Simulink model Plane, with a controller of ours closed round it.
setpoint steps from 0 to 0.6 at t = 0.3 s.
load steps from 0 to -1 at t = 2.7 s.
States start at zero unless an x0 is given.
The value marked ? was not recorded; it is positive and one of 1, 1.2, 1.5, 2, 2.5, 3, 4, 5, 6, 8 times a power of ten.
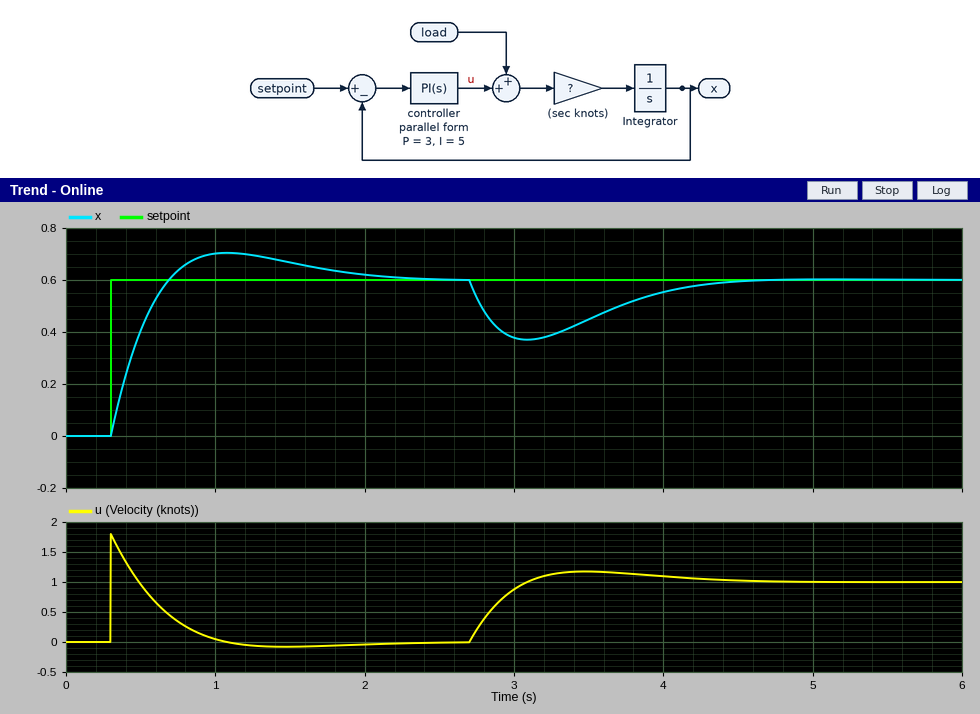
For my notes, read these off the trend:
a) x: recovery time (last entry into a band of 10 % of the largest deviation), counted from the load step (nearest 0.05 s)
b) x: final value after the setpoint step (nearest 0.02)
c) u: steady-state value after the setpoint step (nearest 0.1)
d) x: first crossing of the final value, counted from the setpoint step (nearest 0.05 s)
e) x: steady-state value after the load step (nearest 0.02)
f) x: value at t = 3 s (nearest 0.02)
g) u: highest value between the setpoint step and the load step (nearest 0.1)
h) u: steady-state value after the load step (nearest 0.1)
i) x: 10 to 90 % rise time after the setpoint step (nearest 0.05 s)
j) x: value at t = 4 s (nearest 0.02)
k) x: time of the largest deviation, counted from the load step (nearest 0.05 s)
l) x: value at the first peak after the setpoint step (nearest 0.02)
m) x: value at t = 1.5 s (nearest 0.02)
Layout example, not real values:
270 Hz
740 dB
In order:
1.50 s
0.60
0.0
0.40 s
0.60
0.38
1.8
1.0
0.30 s
0.56
0.40 s
0.70
0.66
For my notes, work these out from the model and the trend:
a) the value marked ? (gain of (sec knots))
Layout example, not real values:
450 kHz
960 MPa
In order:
1.5
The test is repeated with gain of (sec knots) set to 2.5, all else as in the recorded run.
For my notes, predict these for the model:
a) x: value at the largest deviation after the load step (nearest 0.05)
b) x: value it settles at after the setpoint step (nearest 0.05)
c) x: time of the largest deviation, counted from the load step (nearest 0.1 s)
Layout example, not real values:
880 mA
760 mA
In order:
0.35
0.60
0.3 s
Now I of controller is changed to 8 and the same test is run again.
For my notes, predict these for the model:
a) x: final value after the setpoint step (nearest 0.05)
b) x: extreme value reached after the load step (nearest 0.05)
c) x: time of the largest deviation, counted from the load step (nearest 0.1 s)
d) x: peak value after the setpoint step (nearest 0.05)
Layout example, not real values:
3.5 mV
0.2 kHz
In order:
0.60
0.40
0.3 s
0.75
